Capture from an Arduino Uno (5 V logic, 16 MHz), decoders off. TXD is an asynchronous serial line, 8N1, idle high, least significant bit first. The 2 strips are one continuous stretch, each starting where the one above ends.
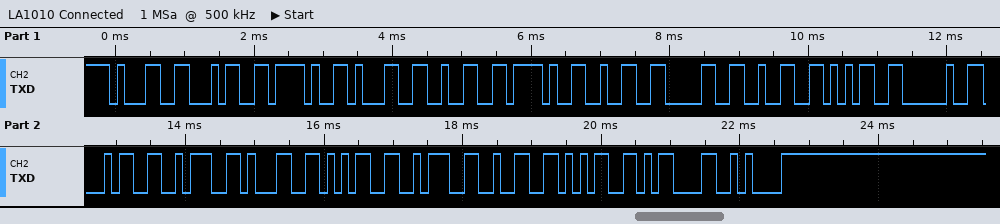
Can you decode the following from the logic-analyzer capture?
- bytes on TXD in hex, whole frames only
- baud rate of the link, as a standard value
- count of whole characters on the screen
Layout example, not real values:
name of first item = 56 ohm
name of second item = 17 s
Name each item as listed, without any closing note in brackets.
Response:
bytes on TXD in hex, whole frames only = 0x31 0x34 0x2F 0x31 0x32 0x2F 0x32 0x30 0x32 0x35 0x20 0x34 0x3A 0x31 0x35 0x3A 0x32 0x35 0x0D 0x0A
baud rate of the link, as a standard value = 9600 baud
count of whole characters on the screen = 20
